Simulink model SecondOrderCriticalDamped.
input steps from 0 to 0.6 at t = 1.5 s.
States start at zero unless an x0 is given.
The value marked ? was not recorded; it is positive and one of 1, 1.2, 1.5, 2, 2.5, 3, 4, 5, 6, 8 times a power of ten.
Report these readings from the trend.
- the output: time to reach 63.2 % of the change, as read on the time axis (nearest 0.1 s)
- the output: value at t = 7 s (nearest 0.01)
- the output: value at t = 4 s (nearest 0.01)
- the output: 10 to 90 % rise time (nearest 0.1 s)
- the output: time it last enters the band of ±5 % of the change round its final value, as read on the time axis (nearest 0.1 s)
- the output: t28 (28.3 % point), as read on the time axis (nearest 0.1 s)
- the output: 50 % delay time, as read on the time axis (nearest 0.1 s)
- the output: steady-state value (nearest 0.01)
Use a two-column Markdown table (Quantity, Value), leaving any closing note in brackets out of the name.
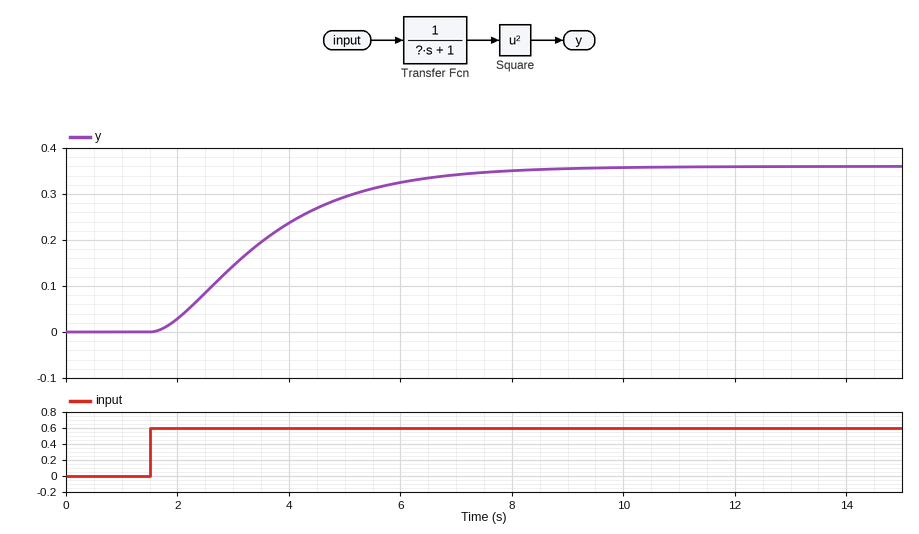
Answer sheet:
| Quantity | Value |
|---|---|
| the output: time to reach 63.2 % of the change, as read on the time axis | 3.9 s |
| the output: value at t = 7 s | 0.34 |
| the output: value at t = 4 s | 0.24 |
| the output: 10 to 90 % rise time | 3.9 s |
| the output: time it last enters the band of ±5 % of the change round its final value, as read on the time axis | 7.0 s |
| the output: t28 (28.3 % point), as read on the time axis | 2.6 s |
| the output: 50 % delay time, as read on the time axis | 3.3 s |
| the output: steady-state value | 0.36 |
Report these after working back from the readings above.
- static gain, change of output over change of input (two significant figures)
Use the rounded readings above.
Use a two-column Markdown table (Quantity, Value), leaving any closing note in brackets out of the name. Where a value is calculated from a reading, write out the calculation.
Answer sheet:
| Quantity | Value |
|---|---|
| static gain, change of output over change of input | (0.36 - 0) / (0.6 - 0) = 0.60 |
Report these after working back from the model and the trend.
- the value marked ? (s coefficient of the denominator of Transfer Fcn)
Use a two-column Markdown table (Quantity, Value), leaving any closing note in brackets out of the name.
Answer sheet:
| Quantity | Value |
|---|---|
| the value marked ? | 1.5 |
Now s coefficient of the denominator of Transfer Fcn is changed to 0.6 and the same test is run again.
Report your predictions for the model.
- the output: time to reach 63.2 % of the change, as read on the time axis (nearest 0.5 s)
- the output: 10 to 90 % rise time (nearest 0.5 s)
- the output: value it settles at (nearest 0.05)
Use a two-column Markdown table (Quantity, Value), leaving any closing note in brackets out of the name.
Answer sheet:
| Quantity | Value |
|---|---|
| the output: time to reach 63.2 % of the change, as read on the time axis | 2.5 s |
| the output: 10 to 90 % rise time | 1.5 s |
| the output: value it settles at | 0.35 |
